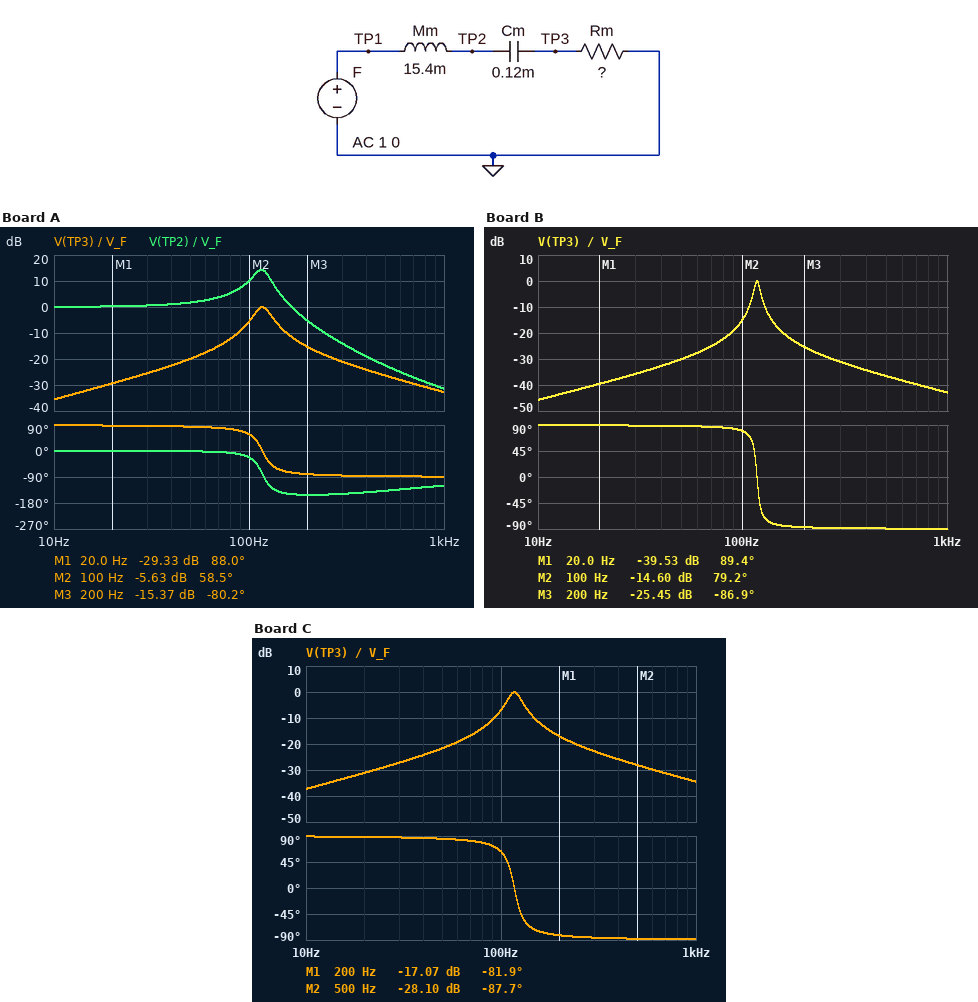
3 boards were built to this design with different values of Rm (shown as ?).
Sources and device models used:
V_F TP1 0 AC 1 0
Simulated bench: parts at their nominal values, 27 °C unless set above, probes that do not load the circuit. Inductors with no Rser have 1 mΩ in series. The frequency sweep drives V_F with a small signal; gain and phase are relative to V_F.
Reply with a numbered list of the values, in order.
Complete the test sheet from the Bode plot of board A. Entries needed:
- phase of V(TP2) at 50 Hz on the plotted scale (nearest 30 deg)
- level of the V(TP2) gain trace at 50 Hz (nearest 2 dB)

1. 0 deg
2. 2 dB
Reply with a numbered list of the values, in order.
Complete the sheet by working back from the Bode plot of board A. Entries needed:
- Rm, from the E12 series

1. 2.2 Ω
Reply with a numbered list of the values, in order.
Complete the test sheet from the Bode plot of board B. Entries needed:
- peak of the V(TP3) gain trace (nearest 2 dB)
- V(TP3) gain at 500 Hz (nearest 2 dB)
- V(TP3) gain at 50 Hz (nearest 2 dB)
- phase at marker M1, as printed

1. 0 dB
2. -36 dB
3. -30 dB
4. 89.4 deg
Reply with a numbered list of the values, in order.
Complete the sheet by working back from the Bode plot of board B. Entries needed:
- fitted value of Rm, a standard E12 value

1. 0.68 Ω
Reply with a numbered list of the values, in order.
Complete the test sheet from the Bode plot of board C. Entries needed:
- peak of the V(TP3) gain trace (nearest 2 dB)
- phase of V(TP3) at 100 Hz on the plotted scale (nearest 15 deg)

1. 0 dB
2. 60 deg
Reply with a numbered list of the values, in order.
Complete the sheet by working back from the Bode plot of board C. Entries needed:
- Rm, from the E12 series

1. 1.8 Ω
